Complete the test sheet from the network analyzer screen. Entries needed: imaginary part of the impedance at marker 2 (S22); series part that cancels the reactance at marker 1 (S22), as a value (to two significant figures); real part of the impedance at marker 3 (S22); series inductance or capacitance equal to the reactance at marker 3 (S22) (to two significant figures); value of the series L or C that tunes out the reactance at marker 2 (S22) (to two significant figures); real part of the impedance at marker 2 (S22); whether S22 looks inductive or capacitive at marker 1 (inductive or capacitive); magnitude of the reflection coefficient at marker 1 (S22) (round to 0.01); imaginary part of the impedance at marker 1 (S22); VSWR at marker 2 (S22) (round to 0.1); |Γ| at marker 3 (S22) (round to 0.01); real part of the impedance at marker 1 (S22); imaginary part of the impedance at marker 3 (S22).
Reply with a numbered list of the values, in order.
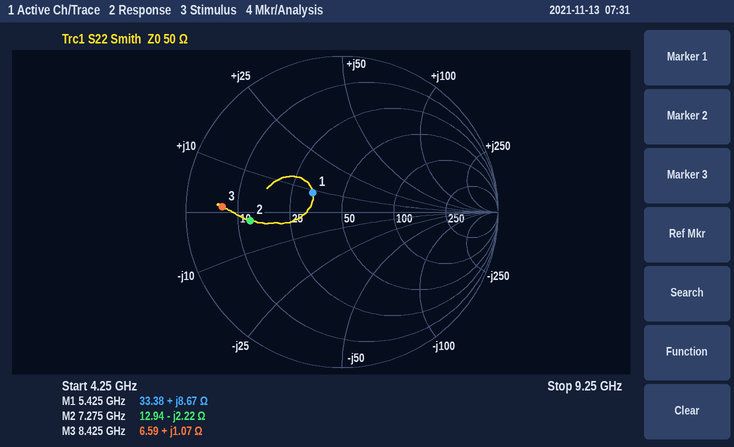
1. -2.22 Ω
2. 3.4 pF
3. 6.59 Ω
4. 20 pH
5. 49 pH
6. 12.94 Ω
7. inductive
8. 0.22
9. +8.67 Ω
10. 3.9
11. 0.77
12. 33.38 Ω
13. +1.07 Ω
